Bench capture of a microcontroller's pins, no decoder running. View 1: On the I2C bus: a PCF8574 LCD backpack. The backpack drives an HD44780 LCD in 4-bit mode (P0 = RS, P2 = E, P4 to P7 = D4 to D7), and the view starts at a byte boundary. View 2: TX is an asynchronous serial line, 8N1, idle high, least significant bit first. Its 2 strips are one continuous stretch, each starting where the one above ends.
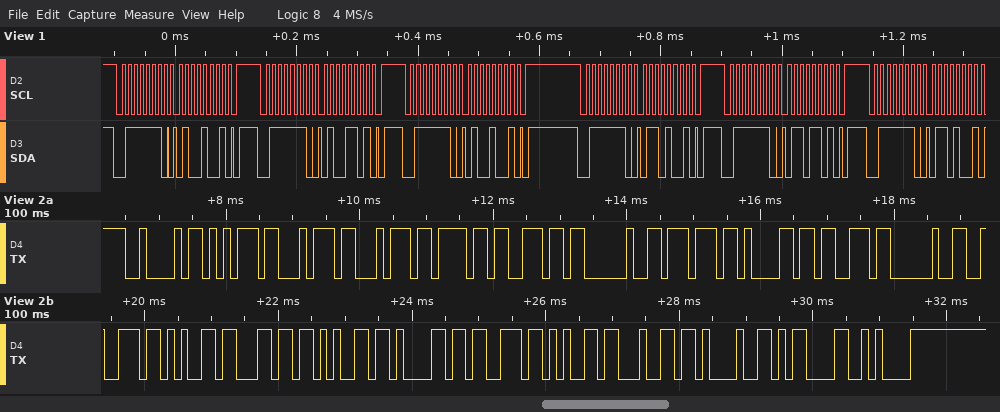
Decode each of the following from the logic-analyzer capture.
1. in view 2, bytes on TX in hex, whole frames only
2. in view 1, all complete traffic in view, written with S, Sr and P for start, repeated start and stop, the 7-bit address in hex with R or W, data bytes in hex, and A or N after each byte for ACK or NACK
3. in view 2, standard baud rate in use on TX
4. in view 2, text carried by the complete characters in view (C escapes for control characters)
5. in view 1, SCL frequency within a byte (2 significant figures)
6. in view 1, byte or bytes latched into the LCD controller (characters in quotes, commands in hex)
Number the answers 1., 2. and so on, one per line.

1. 42 75 74 74 6F 6E 20 77 61 73 20 72 65 6C 65 61 73 65 64 21 0D 0A
2. S 3FW A 49 A P S 3FW A 4D A P S 3FW A 49 A P S 3FW A 69 A P S 3FW A 6D A P S 3FW A 69 A
3. 9600 baud
4. "Button was released!\r\n"
5. 100 kHz
6. 'F'
